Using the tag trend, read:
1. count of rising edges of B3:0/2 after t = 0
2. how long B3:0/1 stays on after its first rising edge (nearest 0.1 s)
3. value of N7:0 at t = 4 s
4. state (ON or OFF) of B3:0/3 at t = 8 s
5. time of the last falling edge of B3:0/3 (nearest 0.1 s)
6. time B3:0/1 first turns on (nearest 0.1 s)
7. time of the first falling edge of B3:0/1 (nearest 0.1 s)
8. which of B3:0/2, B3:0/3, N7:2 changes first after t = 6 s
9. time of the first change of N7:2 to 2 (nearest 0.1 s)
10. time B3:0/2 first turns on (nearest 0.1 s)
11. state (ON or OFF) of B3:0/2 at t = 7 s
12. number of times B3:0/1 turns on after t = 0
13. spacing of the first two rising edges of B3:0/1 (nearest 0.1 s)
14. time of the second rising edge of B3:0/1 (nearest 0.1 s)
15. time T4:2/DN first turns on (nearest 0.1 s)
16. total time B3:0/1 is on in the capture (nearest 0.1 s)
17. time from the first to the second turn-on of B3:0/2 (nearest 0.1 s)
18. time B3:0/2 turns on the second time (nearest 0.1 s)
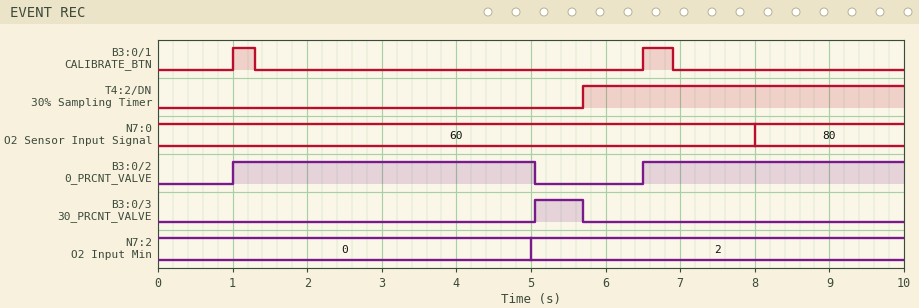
2
0.3 s
60
OFF
5.7 s
1.0 s
1.3 s
B3:0/2
5.0 s
1.0 s
ON
2
5.5 s
6.5 s
5.7 s
0.7 s
5.5 s
6.5 s
